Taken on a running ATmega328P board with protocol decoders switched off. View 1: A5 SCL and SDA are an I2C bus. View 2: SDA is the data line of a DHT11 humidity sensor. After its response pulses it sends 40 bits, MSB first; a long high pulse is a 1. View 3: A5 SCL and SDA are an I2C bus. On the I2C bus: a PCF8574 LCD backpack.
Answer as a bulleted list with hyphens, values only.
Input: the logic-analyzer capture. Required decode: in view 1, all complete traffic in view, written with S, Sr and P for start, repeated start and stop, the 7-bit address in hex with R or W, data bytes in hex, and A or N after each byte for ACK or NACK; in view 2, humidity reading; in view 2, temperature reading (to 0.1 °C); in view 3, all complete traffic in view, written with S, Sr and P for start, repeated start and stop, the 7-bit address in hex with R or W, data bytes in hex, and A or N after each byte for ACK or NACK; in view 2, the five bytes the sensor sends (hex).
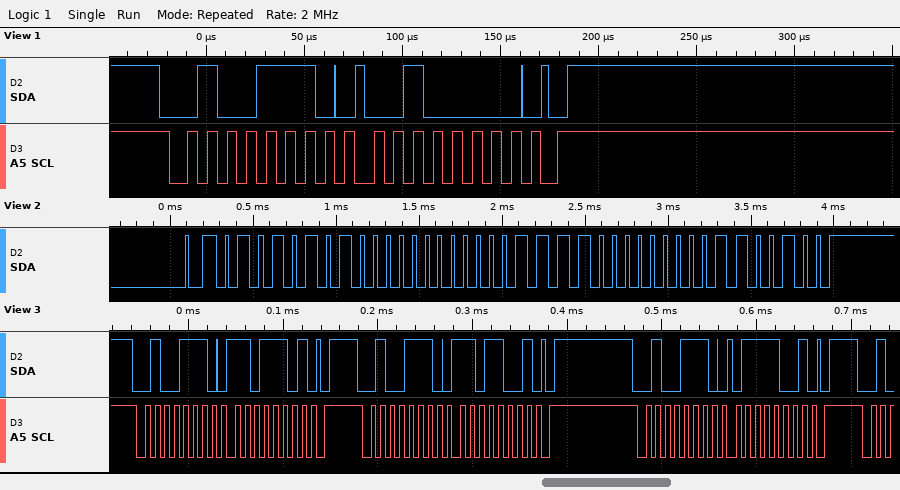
- S 27W A 20 A P
- 85 %
- 15.0 °C
- S 27W A DD A P S 27W A D9 A P S 27W A 79 A P
- 55 00 0F 00 64
